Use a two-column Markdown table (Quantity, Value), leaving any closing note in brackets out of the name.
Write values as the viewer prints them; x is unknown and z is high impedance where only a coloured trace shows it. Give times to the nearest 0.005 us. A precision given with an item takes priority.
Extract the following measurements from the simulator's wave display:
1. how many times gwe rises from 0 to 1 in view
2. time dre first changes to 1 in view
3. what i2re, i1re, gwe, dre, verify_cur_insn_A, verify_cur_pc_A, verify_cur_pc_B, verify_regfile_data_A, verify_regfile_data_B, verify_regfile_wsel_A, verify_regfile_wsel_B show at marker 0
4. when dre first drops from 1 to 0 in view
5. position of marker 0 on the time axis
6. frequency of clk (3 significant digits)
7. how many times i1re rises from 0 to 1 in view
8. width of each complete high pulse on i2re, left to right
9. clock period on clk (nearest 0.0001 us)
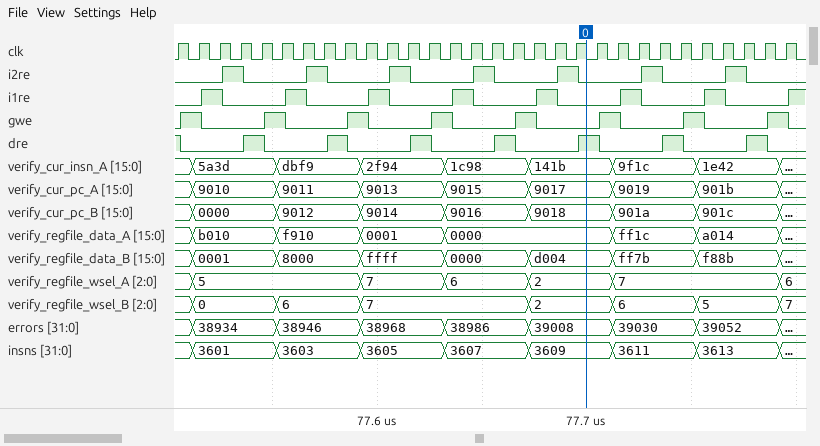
| Quantity | Value |
|---|---|
| how many times gwe rises from 0 to 1 in view | 8 |
| time dre first changes to 1 in view | 77.535 us |
| what i2re, i1re, gwe, dre, verify_cur_insn_A, verify_cur_pc_A, verify_cur_pc_B, verify_regfile_data_A, verify_regfile_data_B, verify_regfile_wsel_A, verify_regfile_wsel_B show at marker 0 | i2re=0, i1re=0, gwe=0, dre=1, verify_cur_insn_A=141b, verify_cur_pc_A=9017, verify_cur_pc_B=9018, verify_regfile_data_A=0000, verify_regfile_data_B=d004, verify_regfile_wsel_A=2, verify_regfile_wsel_B=2 |
| when dre first drops from 1 to 0 in view | 77.505 us |
| position of marker 0 on the time axis | 77.7 us |
| frequency of clk | 100 MHz |
| how many times i1re rises from 0 to 1 in view | 8 |
| width of each complete high pulse on i2re, left to right | 0.01 us, 0.01 us, 0.01 us, 0.01 us, 0.01 us, 0.01 us, 0.01 us |
| clock period on clk | 0.01 us |
